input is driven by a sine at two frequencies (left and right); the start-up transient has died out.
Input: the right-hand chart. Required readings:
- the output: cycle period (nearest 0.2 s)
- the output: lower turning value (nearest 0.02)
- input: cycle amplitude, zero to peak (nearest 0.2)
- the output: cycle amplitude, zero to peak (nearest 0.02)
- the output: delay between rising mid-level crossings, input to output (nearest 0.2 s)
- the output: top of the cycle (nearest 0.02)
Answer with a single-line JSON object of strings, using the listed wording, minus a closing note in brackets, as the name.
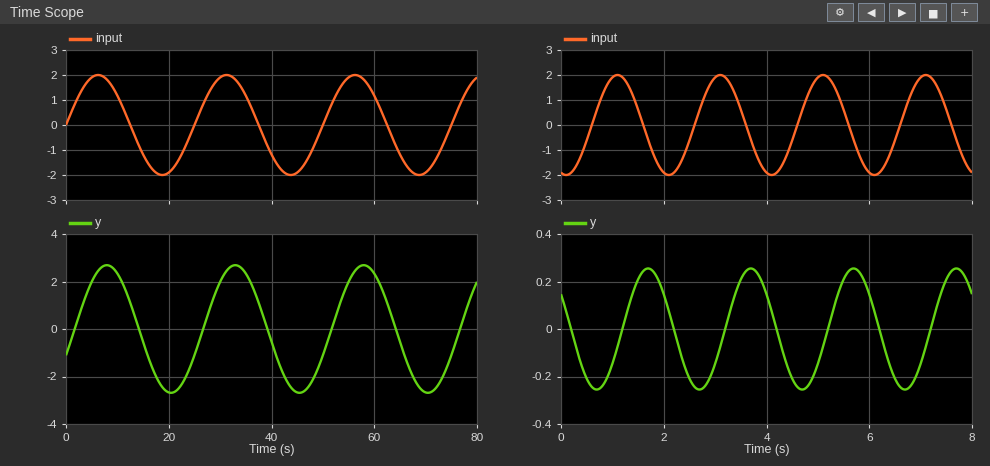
{"the output: cycle period": "2.0 s", "the output: lower turning value": "-0.26", "input: cycle amplitude, zero to peak": "2.0", "the output: cycle amplitude, zero to peak": "0.26", "the output: delay between rising mid-level crossings, input to output": "0.6 s", "the output: top of the cycle": "0.26"}
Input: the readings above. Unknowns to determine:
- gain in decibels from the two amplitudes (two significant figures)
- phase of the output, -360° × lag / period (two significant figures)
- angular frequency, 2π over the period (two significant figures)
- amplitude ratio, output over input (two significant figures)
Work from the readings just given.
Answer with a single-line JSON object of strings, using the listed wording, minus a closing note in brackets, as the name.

{"gain in decibels from the two amplitudes": "-18 dB", "phase of the output, -360° × lag / period": "-110°", "angular frequency, 2π over the period": "3.1 rad/s", "amplitude ratio, output over input": "0.13"}
